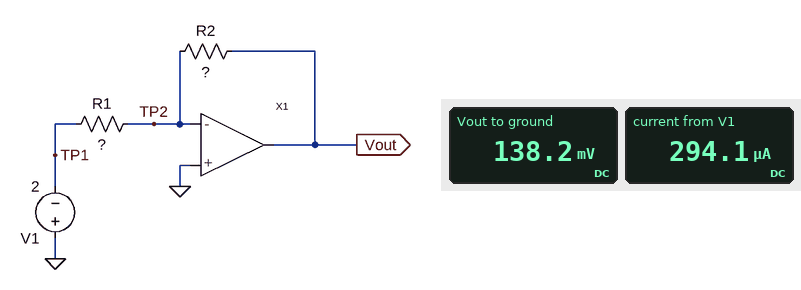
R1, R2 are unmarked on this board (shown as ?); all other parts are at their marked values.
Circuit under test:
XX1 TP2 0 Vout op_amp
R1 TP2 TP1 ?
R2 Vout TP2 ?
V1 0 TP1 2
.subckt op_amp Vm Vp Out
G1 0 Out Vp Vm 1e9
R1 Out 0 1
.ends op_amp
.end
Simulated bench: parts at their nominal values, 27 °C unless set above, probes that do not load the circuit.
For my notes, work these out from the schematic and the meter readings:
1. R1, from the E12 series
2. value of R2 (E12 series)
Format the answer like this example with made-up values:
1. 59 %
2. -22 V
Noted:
1. 6.8 kΩ
2. 470 Ω
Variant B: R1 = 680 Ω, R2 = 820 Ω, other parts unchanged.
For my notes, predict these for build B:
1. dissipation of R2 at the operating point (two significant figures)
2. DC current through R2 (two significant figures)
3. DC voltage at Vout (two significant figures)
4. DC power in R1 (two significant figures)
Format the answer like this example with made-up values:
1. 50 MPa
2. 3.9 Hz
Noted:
1. 7.1 mW
2. 2.9 mA
3. 2.4 V
4. 5.9 mW
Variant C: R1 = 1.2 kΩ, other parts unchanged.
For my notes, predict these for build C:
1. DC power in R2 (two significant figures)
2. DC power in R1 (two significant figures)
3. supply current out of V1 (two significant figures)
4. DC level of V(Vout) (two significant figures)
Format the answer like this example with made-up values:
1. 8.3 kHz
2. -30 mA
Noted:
1. 1.3 mW
2. 3.3 mW
3. 1.7 mA
4. 780 mV
